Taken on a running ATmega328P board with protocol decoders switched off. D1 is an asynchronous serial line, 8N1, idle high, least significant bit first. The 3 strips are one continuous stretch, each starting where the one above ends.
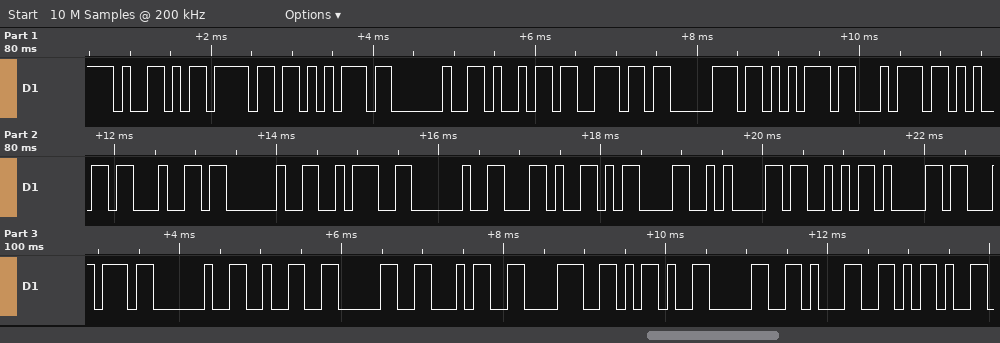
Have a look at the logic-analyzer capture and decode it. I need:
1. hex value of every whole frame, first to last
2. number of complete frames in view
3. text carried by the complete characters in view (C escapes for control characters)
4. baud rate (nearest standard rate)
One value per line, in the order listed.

0x59 0x6F 0x75 0x20 0x69 0x6E 0x70 0x75 0x74 0x65 0x64 0x20 0x3A 0x20 0x2C 0x0D 0x0A 0x53 0x61 0x74 0x20 0x32 0x30 0x34 0x38 0x2D 0x30 0x31 0x2D
29
"You inputed : ,\r\nSat 2048-01-"
9600 baud
